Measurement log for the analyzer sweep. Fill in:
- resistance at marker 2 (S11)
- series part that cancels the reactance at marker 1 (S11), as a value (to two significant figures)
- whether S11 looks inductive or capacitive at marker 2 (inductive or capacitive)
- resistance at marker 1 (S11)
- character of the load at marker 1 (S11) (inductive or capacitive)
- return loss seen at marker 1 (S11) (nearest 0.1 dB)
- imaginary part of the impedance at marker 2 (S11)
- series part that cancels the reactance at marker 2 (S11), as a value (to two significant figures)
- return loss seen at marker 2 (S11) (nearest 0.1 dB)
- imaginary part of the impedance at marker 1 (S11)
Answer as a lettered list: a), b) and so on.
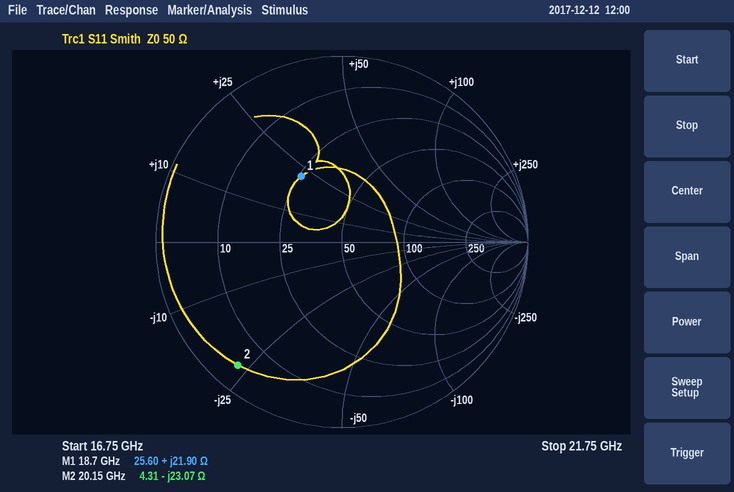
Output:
a) 4.31 Ω
b) 390 fF
c) capacitive
d) 25.60 Ω
e) inductive
f) 7.6 dB
g) -23.07 Ω
h) 180 pH
i) 1.2 dB
j) +21.90 Ω
